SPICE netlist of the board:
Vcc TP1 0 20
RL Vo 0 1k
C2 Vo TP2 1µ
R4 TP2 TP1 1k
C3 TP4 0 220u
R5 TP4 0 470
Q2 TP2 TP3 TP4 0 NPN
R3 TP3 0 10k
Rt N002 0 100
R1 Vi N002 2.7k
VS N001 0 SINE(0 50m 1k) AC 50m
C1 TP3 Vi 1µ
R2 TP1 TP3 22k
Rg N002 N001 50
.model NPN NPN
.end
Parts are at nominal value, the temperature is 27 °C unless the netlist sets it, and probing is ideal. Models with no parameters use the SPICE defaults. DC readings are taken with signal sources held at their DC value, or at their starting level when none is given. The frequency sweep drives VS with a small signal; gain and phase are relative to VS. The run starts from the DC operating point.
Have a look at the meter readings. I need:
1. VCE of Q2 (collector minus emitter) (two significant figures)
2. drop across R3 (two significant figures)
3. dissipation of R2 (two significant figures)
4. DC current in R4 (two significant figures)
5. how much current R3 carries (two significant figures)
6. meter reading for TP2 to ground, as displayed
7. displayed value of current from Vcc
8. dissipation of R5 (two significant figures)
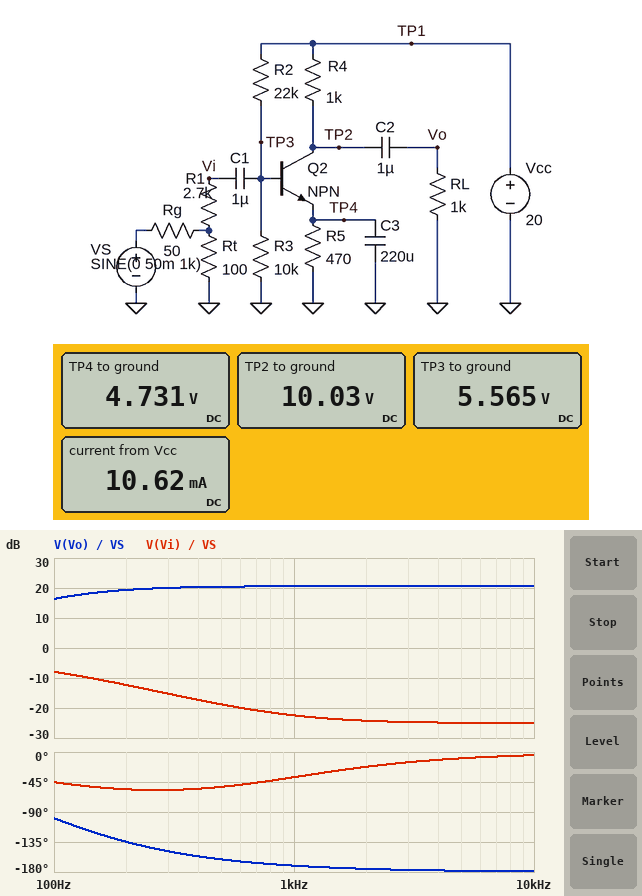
5.3 V
5.6 V
9.5 mW
10 mA
560 µA
10.03 V
10.62 mA
48 mW
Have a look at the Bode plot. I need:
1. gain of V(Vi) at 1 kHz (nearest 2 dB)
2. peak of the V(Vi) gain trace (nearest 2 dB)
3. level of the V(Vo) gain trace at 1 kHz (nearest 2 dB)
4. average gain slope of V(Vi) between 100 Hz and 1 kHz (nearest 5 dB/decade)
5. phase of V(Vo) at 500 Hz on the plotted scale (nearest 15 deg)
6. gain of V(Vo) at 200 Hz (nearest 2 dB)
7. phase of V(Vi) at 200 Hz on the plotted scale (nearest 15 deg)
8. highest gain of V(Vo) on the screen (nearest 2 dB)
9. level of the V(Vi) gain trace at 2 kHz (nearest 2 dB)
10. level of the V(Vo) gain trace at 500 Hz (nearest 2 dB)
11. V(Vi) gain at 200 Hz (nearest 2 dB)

-22 dB
-8 dB
20 dB
-15 dB/decade
-165 deg
20 dB
-60 deg
20 dB
-24 dB
20 dB
-12 dB
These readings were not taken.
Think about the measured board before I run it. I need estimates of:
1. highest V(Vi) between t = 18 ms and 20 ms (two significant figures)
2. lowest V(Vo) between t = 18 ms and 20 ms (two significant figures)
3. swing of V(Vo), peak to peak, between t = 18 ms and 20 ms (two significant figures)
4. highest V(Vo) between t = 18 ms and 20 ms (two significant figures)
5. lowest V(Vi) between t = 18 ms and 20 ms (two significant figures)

3.8 mV
-540 mV
1.1 V
530 mV
-3.8 mV
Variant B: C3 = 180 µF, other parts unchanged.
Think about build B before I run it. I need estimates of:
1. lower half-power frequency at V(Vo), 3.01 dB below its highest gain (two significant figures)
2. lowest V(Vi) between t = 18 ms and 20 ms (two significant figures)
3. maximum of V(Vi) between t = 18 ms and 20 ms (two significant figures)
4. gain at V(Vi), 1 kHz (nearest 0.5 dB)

130 Hz
-3.9 mV
3.9 mV
-22.0 dB
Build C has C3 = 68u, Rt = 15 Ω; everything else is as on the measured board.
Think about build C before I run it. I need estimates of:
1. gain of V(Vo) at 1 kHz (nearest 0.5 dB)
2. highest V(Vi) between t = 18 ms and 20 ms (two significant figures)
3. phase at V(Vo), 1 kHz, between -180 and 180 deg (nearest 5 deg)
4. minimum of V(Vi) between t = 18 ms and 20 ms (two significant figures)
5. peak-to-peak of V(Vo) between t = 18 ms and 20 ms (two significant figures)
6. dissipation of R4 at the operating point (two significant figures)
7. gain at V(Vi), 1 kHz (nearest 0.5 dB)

11.5 dB
1.8 mV
-165 deg
-1.8 mV
370 mV
99 mW
-29.0 dB
